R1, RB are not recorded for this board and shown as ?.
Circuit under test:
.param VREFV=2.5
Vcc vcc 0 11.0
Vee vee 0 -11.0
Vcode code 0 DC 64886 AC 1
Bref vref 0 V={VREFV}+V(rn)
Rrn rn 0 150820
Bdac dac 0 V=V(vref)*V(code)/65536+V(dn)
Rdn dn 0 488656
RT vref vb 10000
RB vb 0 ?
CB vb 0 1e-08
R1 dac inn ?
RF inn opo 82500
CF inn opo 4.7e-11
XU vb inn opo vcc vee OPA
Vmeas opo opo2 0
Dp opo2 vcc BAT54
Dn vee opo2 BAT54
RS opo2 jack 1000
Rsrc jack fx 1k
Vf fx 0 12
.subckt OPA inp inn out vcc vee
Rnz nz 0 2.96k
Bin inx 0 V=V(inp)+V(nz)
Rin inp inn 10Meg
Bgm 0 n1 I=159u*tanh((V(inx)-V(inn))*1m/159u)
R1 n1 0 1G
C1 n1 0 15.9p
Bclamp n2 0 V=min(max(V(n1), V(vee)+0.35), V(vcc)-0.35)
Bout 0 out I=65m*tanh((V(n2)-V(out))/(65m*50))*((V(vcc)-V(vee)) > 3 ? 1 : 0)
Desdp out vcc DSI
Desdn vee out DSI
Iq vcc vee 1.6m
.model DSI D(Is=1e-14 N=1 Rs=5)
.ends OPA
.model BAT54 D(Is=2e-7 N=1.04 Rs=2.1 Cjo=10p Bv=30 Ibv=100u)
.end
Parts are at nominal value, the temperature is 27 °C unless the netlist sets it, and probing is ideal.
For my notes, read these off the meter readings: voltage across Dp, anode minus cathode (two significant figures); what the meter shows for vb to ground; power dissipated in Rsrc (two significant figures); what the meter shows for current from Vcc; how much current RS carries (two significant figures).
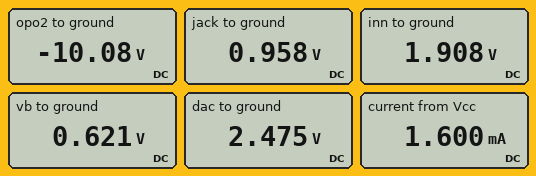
-21 V
0.621 V
120 mW
1.600 mA
11 mA
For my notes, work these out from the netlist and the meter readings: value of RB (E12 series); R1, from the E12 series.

3.3 kΩ
3.9 kΩ
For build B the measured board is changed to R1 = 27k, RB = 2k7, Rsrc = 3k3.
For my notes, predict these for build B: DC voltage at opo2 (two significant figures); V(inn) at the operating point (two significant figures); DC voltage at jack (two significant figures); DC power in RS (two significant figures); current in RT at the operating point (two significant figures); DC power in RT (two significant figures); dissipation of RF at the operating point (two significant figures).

-5.4 V
530 mV
-1.4 V
16 mW
200 µA
390 µW
430 µW
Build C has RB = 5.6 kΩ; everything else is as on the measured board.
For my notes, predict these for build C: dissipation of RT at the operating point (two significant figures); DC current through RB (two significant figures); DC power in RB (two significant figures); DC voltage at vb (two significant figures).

260 µW
160 µA
140 µW
900 mV
